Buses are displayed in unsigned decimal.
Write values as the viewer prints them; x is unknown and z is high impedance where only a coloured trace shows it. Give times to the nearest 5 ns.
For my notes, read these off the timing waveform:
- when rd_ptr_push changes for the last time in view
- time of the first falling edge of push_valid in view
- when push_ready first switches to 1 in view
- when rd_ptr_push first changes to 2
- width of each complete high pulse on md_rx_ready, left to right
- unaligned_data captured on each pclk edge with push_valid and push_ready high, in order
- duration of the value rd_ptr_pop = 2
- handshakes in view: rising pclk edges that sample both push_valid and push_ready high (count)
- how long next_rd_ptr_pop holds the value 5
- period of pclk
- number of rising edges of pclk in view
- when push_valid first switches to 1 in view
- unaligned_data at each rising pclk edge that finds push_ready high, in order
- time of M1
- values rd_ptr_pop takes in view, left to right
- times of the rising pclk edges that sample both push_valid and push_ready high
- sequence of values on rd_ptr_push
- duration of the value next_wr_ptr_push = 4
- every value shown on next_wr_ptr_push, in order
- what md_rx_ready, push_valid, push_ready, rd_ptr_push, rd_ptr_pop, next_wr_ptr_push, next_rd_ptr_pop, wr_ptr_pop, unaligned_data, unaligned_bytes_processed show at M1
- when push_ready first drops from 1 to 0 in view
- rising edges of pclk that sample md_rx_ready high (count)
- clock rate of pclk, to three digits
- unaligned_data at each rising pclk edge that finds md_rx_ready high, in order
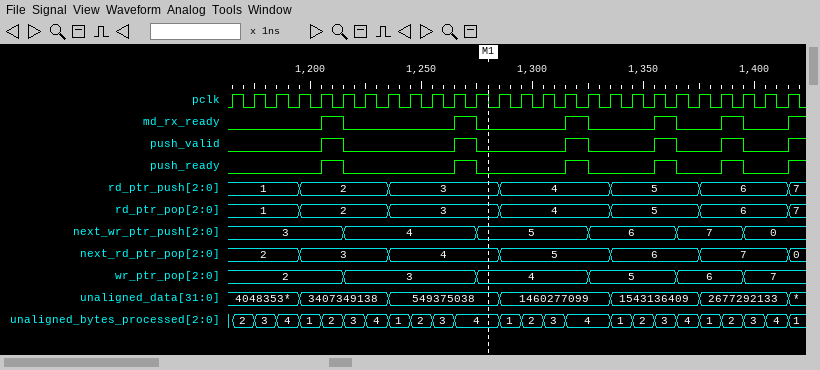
1415 ns
1215 ns
1205 ns
1195 ns
10 ns, 10 ns, 10 ns, 10 ns, 10 ns
3407349138, 549375038, 1460277099, 1543136409, 2677292133
40 ns
5
50 ns
10 ns
26
1205 ns
3407349138, 549375038, 1460277099, 1543136409, 2677292133
1280 ns
1, 2, 3, 4, 5, 6, 7
1215 ns, 1275 ns, 1325 ns, 1365 ns, 1395 ns
1, 2, 3, 4, 5, 6, 7
60 ns
3, 4, 5, 6, 7, 0
md_rx_ready=0, push_valid=0, push_ready=0, rd_ptr_push=3, rd_ptr_pop=3, next_wr_ptr_push=5, next_rd_ptr_pop=4, wr_ptr_pop=4, unaligned_data=549375038, unaligned_bytes_processed=4
1215 ns
5
100 MHz
3407349138, 549375038, 1460277099, 1543136409, 2677292133
